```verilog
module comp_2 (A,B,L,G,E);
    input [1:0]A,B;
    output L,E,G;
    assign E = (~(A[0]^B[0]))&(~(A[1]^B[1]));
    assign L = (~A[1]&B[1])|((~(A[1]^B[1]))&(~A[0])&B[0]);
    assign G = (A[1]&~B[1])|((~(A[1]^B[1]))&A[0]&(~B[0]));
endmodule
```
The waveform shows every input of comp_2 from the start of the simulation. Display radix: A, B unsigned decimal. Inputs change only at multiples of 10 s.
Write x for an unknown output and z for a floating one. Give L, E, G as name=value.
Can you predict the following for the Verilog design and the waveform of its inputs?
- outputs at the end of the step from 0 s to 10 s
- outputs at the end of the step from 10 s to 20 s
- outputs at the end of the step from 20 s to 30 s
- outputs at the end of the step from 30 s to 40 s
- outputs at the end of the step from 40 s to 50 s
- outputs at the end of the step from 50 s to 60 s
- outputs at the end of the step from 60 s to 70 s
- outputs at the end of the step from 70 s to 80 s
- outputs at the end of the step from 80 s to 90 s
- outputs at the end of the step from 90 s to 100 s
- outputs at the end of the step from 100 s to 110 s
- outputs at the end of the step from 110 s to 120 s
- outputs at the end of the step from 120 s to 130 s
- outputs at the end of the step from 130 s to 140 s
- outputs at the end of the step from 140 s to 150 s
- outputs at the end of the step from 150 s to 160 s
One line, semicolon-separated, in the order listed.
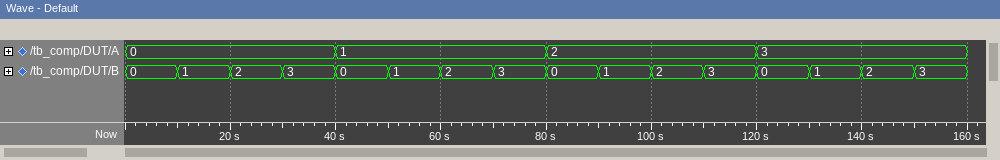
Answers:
L=0, E=1, G=0; L=1, E=0, G=0; L=1, E=0, G=0; L=1, E=0, G=0; L=0, E=0, G=1; L=0, E=1, G=0; L=1, E=0, G=0; L=1, E=0, G=0; L=0, E=0, G=1; L=0, E=0, G=1; L=0, E=1, G=0; L=1, E=0, G=0; L=0, E=0, G=1; L=0, E=0, G=1; L=0, E=0, G=1; L=0, E=1, G=0
